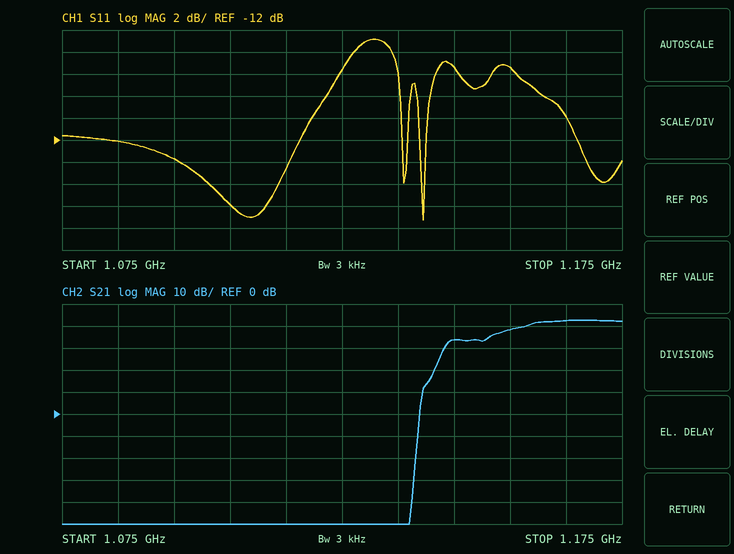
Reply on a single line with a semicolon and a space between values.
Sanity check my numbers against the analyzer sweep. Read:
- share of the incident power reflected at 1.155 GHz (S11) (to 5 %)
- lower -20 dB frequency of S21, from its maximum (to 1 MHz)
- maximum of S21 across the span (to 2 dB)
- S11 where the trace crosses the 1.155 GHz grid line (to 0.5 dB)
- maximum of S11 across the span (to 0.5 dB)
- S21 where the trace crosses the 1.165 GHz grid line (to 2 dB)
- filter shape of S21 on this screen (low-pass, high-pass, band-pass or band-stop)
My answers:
30 %; 1.142 GHz; 42 dB; -5.5 dB; -3.0 dB; 42 dB; high-pass
